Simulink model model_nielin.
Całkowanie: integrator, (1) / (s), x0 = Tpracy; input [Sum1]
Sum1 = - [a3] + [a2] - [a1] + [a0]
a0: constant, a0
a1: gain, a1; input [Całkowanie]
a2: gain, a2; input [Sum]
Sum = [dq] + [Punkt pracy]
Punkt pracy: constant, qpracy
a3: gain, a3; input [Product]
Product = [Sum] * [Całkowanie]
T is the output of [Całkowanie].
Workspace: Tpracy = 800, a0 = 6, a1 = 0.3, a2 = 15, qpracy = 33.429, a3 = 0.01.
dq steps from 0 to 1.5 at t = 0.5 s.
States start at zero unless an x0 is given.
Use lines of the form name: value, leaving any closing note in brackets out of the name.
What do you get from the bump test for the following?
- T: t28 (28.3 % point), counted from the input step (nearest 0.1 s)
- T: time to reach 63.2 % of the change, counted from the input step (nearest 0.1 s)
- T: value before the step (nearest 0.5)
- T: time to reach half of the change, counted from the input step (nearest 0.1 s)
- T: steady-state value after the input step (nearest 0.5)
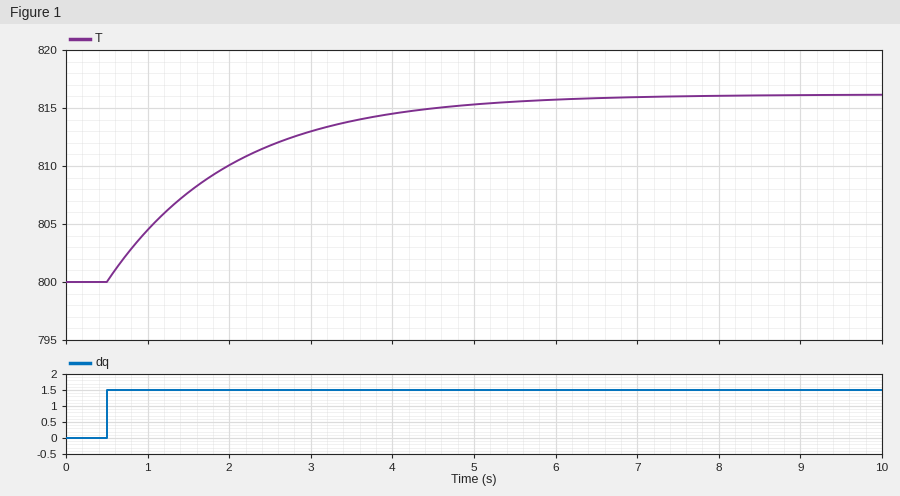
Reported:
T: t28 (28.3 % point), counted from the input step: 0.5 s
T: time to reach 63.2 % of the change, counted from the input step: 1.5 s
T: value before the step: 800.0
T: time to reach half of the change, counted from the input step: 1.1 s
T: steady-state value after the input step: 816.0
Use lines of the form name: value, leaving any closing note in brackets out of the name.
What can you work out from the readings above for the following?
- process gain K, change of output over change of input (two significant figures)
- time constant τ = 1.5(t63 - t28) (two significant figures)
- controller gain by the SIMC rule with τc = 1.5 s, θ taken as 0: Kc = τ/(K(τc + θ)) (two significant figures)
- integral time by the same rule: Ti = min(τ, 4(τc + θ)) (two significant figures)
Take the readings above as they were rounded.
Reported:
process gain K, change of output over change of input: 11
time constant τ = 1.5(t63 - t28): 1.5 s
controller gain by the SIMC rule with τc = 1.5 s, θ taken as 0: Kc = τ/(K(τc + θ)): 0.091
integral time by the same rule: Ti = min(τ, 4(τc + θ)): 1.5 s
